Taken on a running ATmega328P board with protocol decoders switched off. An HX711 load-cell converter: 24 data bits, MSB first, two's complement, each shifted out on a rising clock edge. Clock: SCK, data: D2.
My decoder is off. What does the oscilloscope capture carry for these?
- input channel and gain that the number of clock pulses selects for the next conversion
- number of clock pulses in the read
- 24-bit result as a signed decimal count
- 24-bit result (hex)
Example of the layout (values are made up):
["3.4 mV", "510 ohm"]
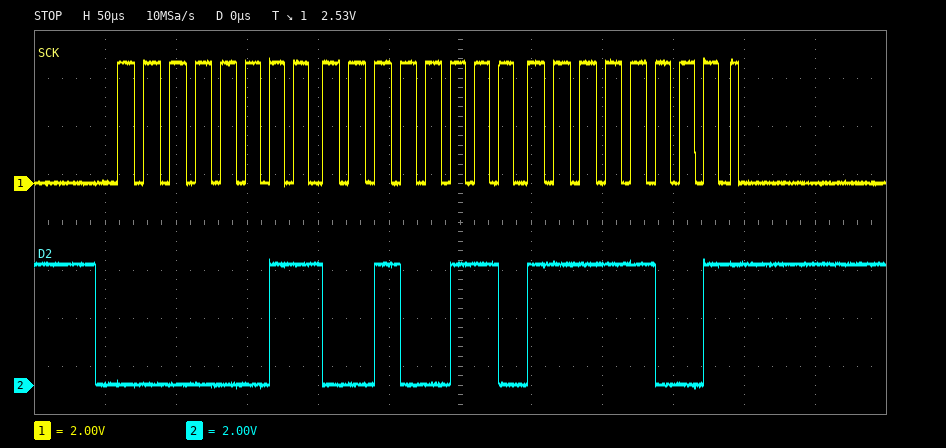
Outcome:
["channel A, gain 128", "25", "206585", "0x0326F9"]
